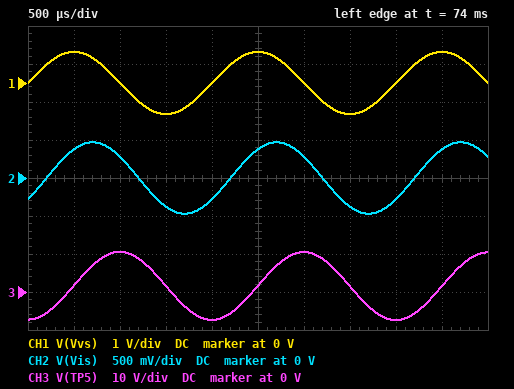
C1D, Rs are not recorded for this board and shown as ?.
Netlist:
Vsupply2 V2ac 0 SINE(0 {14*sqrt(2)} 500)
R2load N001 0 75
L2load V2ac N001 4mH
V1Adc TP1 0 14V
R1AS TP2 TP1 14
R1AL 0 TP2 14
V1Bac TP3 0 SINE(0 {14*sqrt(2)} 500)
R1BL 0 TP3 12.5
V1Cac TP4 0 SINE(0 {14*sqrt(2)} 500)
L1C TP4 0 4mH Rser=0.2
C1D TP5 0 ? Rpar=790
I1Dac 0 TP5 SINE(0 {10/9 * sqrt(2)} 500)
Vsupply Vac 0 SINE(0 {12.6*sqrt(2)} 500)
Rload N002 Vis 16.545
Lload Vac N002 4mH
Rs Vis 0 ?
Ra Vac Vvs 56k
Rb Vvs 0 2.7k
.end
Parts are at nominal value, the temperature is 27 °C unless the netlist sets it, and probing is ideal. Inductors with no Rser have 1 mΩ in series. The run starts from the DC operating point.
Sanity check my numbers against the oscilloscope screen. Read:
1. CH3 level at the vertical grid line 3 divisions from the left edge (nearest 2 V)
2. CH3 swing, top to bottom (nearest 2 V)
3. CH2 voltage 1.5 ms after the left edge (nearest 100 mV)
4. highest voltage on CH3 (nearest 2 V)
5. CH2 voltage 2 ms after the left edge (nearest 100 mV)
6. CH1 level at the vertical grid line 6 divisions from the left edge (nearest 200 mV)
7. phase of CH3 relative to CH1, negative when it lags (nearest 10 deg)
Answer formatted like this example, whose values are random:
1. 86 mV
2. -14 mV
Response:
1. 2 V
2. 18 V
3. -400 mV
4. 10 V
5. -300 mV
6. 0 V
7. -90 deg
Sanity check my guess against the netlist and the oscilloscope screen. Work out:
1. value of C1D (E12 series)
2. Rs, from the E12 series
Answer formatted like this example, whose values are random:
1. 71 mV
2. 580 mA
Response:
1. 56 µF
2. 0.56 Ω
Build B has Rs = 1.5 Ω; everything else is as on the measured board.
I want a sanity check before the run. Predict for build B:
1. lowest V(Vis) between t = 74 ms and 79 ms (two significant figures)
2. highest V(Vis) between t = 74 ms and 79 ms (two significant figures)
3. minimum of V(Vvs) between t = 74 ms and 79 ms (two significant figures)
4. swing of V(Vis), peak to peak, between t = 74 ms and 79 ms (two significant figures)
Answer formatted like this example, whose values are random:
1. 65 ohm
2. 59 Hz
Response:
1. -1.2 V
2. 1.2 V
3. -820 mV
4. 2.4 V
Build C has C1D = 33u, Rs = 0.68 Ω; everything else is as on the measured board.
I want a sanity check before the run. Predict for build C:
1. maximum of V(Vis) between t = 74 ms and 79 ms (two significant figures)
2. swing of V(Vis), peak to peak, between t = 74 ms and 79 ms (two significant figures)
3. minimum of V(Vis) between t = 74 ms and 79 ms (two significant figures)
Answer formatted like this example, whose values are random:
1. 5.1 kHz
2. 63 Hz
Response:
1. 570 mV
2. 1.1 V
3. -570 mV
